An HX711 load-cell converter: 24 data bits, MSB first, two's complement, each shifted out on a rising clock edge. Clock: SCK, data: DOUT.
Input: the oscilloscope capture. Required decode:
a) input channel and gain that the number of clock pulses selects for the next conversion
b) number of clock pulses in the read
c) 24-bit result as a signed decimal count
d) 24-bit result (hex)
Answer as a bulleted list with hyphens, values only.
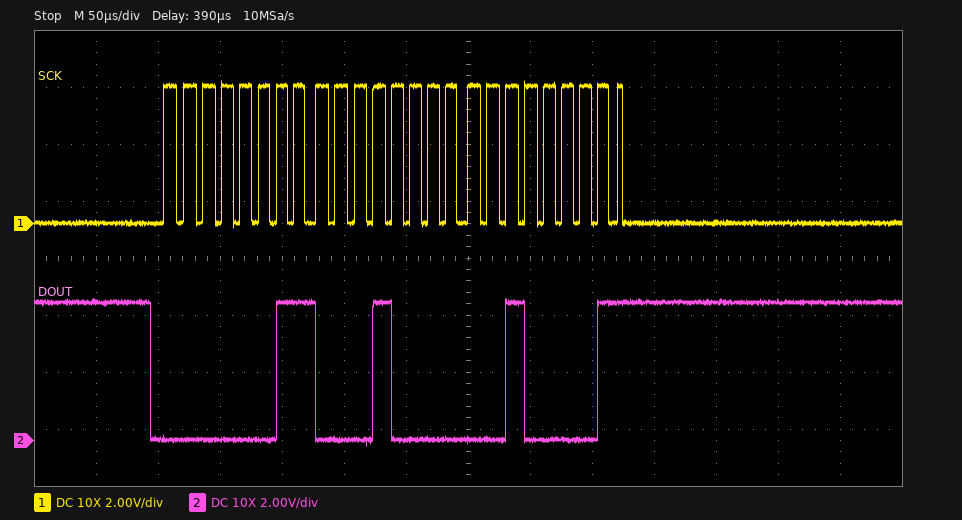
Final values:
- channel A, gain 128
- 25
- 200737
- 0x031021
